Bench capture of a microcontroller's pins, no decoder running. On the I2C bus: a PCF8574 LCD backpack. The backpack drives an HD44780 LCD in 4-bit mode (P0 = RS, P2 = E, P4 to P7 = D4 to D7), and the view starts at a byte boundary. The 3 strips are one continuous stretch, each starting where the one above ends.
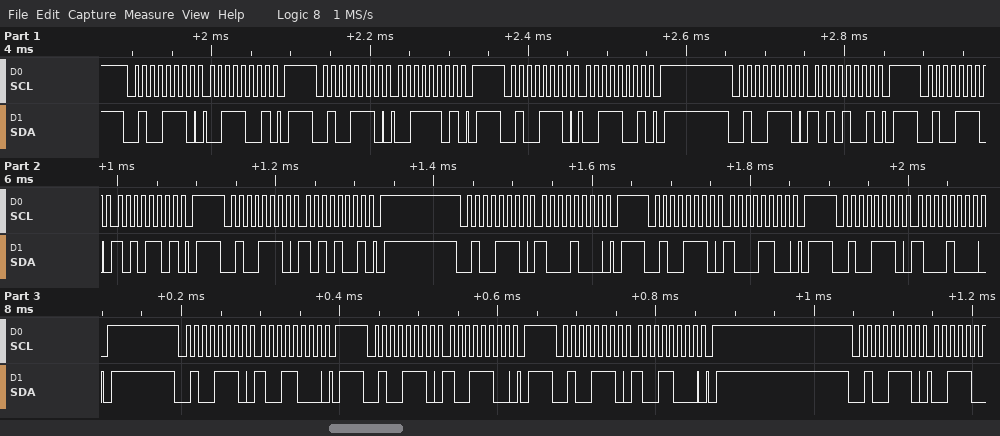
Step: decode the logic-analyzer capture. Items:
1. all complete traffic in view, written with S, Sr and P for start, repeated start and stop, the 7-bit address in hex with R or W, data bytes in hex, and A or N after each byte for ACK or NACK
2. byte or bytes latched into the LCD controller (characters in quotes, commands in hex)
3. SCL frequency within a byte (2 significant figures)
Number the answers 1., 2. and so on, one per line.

1. S 27W A 39 A P S 27W A 3D A P S 27W A 39 A P S 27W A A9 A P S 27W A AD A P S 27W A A9 A P S 27W A 88 A P S 27W A 8C A P S 27W A 88 A P S 27W A 98 A P S 27W A 9C A P S 27W A 98 A P S 27W A
2. ':' 0x89
3. 100 kHz
